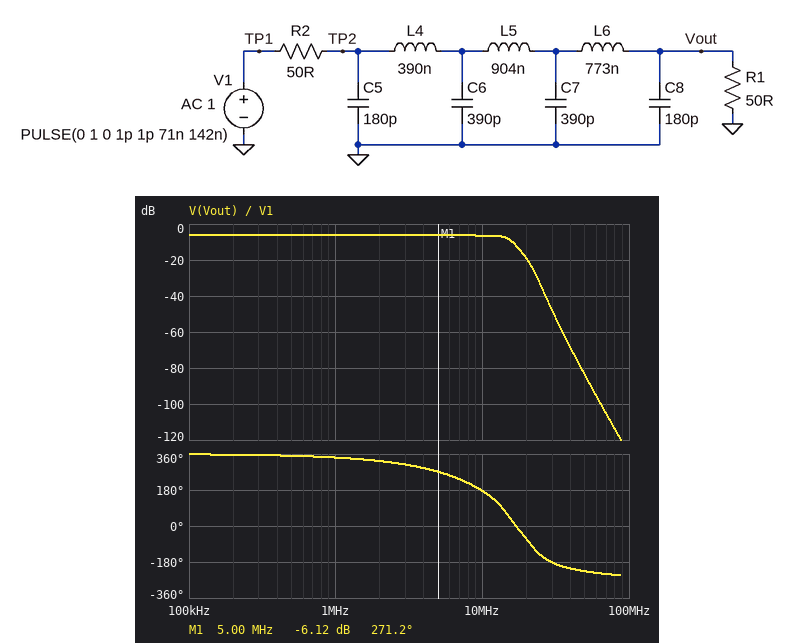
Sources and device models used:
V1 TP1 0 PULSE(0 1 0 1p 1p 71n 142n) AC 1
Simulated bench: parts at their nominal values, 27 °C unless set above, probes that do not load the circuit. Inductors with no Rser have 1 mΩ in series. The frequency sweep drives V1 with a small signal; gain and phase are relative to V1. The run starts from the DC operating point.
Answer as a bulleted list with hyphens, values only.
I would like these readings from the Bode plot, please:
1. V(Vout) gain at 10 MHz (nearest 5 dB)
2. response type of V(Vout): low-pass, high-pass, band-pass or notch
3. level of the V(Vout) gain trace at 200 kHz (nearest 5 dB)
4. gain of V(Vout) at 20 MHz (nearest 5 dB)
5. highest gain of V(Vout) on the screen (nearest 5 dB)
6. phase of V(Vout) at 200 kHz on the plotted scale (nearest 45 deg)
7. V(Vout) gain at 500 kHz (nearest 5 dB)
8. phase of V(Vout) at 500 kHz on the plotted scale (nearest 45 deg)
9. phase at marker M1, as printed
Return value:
- -5 dB
- low-pass
- -5 dB
- -20 dB
- -5 dB
- 360 deg
- -5 dB
- 360 deg
- 271.2 deg
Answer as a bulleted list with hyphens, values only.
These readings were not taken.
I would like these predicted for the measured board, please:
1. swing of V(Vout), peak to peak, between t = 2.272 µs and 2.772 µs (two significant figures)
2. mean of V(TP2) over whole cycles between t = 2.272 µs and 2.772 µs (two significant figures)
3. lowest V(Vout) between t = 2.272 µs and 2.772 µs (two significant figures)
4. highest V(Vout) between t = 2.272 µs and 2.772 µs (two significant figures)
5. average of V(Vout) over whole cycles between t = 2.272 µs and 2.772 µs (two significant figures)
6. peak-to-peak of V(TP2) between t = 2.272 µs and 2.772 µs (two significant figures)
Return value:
- 620 mV
- 250 mV
- -60 mV
- 560 mV
- 250 mV
- 770 mV
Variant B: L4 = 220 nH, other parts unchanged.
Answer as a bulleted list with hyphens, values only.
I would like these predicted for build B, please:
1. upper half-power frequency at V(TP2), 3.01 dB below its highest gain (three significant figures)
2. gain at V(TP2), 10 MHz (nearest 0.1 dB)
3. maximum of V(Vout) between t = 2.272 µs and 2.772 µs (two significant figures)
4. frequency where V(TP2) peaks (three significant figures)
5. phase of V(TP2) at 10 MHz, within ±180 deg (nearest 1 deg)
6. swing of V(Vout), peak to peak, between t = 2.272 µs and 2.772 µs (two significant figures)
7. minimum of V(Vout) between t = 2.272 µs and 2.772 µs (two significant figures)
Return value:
- 38.6 MHz
- -7.3 dB
- 550 mV
- 31.0 MHz
- -26 deg
- 590 mV
- -47 mV
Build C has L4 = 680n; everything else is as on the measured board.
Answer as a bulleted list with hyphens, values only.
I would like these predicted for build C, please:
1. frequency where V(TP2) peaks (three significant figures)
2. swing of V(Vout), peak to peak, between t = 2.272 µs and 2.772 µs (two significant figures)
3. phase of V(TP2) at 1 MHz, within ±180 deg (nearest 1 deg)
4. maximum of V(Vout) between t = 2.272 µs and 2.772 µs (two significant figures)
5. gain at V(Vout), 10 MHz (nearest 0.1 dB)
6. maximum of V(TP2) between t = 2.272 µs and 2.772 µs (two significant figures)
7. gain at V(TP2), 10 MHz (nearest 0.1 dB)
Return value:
- 18.8 MHz
- 640 mV
- -2 deg
- 570 mV
- -6.1 dB
- 650 mV
- -6.6 dB
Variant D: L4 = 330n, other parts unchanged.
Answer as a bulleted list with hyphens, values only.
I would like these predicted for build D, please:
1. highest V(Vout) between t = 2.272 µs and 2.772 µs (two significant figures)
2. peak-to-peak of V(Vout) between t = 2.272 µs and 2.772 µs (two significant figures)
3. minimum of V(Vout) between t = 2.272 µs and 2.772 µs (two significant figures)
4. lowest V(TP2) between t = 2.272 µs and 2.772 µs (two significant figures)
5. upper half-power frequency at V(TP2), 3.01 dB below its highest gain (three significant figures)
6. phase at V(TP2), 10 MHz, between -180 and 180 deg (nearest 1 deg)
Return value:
- 550 mV
- 610 mV
- -53 mV
- -140 mV
- 33.4 MHz
- -21 deg
